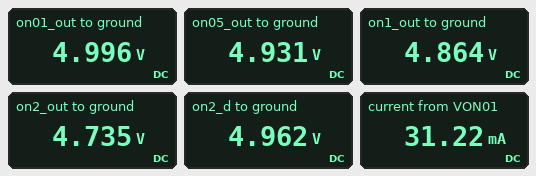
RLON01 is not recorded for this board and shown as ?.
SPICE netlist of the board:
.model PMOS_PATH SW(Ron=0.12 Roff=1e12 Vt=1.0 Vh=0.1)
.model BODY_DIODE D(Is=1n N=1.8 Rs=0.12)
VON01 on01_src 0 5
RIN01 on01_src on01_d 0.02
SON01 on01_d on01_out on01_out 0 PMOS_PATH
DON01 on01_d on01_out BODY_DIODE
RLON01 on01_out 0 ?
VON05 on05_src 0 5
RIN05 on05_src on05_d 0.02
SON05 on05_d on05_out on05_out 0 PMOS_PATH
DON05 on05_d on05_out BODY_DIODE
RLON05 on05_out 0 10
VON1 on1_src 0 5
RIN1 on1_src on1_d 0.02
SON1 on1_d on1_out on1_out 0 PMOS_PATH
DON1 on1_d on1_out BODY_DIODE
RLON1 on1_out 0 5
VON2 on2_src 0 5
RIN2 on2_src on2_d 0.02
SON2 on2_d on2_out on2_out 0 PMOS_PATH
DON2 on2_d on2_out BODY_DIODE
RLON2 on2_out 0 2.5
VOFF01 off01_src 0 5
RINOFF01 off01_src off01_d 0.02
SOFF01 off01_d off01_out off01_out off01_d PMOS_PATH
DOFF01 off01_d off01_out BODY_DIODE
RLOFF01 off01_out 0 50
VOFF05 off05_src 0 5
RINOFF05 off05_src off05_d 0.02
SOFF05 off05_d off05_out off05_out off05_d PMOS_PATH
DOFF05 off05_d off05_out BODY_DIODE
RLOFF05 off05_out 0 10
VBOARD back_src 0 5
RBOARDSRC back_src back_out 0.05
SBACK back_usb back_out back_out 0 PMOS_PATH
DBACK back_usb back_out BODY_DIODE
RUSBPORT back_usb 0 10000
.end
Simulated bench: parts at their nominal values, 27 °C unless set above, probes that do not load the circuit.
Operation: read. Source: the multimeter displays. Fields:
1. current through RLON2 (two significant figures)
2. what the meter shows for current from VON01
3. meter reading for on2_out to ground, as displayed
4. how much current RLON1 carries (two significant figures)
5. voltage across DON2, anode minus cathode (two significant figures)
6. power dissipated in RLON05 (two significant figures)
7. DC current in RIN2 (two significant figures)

1.9 A
31.22 mA
4.735 V
970 mA
230 mV
2.4 W
1.9 A
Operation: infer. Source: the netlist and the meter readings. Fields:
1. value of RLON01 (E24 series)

160 Ω
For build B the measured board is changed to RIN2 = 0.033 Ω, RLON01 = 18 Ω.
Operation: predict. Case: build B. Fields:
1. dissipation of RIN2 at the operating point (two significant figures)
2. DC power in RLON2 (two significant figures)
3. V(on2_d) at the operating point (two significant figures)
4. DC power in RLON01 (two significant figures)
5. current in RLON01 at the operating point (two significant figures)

120 mW
8.9 W
4.9 V
1.4 W
280 mA
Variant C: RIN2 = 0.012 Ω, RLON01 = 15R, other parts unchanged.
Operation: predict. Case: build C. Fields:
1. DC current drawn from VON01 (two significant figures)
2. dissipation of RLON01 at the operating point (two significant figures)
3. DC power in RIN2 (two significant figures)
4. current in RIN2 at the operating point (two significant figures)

330 mA
1.6 W
43 mW
1.9 A
